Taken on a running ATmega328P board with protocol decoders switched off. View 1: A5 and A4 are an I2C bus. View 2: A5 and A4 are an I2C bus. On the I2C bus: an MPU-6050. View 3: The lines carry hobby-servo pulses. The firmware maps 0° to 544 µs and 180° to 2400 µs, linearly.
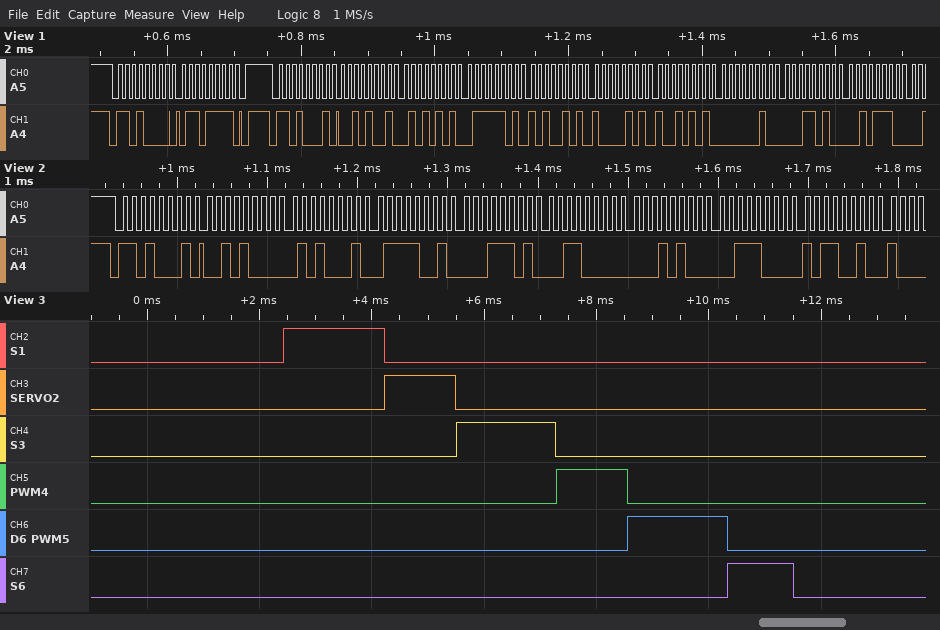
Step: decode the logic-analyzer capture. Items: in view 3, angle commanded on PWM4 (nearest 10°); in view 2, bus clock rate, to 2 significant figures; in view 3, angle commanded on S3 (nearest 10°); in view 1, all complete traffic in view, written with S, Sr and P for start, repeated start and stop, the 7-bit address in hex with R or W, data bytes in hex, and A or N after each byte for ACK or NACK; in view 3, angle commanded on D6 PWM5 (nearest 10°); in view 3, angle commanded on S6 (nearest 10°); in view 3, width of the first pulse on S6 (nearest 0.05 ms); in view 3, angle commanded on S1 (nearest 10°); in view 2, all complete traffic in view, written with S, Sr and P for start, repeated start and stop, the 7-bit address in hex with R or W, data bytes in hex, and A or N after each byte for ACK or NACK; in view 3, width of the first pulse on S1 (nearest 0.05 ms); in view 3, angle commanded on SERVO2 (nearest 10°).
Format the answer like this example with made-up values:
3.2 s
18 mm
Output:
70°
100 kHz
120°
S 68W A 6F A P S 68R A 29 A 55 A 7D A A5 A 85 A 95 A 02 A 1A A 2E A
120°
60°
1.15 ms
120°
S 68R A 28 A 51 A 79 A 1D A 30 A 14 A 38 A B2 A
1.80 ms
70°
